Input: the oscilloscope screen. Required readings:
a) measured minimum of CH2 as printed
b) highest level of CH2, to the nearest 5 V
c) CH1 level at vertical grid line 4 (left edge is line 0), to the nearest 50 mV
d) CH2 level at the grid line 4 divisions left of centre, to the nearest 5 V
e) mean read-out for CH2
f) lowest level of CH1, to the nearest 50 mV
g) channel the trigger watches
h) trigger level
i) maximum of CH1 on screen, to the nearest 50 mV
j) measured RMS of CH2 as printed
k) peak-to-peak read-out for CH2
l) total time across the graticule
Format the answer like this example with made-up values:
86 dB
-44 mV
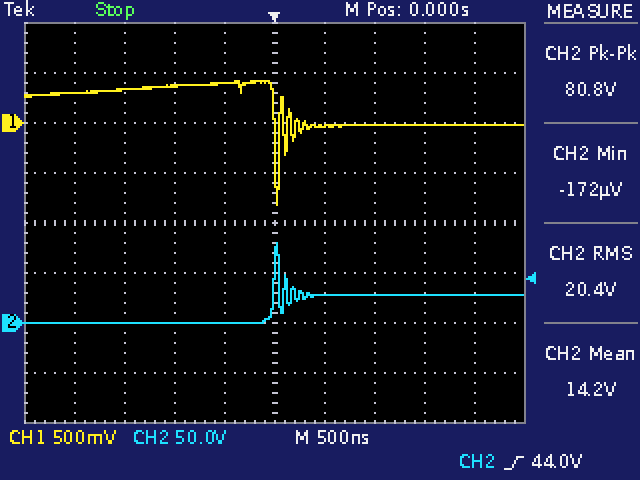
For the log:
-172 µV
80 V
400 mV
0 V
14.2 V
-800 mV
CH2
44.0 V
400 mV
20.4 V
80.8 V
5 µs
